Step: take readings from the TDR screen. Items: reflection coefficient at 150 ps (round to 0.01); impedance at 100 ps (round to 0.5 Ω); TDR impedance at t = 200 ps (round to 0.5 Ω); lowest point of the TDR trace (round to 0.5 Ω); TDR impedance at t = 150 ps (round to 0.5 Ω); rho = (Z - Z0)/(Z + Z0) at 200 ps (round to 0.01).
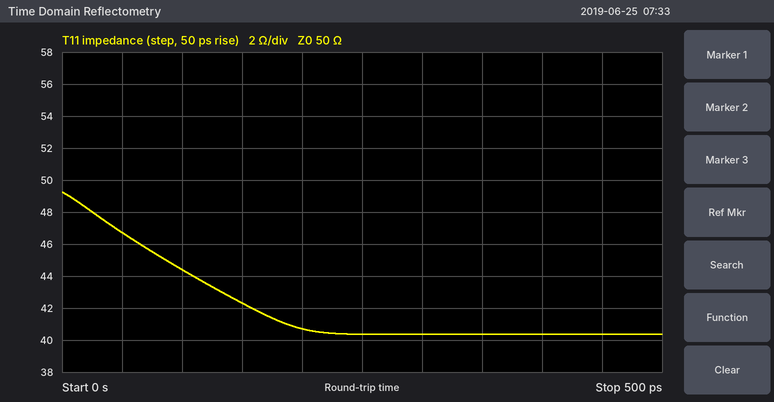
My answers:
-0.08
44.5 Ω
40.5 Ω
40.5 Ω
42.5 Ω
-0.10
